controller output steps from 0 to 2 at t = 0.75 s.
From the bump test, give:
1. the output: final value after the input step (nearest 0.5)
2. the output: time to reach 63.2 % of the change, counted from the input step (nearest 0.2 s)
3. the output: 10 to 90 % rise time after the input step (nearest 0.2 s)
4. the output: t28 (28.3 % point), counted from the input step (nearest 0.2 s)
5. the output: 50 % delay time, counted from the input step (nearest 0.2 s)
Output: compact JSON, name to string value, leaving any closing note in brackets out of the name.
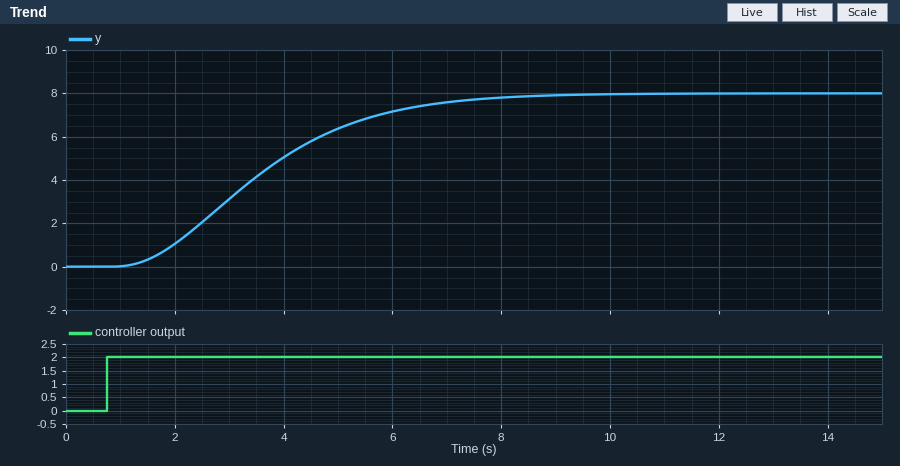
{"the output: final value after the input step": "8.0", "the output: time to reach 63.2 % of the change, counted from the input step": "3.2 s", "the output: 10 to 90 % rise time after the input step": "4.2 s", "the output: t28 (28.3 % point), counted from the input step": "1.8 s", "the output: 50 % delay time, counted from the input step": "2.6 s"}
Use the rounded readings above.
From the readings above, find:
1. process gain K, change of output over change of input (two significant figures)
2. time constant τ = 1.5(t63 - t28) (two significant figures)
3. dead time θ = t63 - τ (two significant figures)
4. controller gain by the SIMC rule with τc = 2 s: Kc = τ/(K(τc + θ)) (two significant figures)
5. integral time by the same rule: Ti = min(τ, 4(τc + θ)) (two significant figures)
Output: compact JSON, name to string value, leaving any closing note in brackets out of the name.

{"process gain K, change of output over change of input": "4.0", "time constant τ = 1.5(t63 - t28)": "2.1 s", "dead time θ = t63 - τ": "1.1 s", "controller gain by the SIMC rule with τc = 2 s: Kc = τ/(K(τc + θ))": "0.17", "integral time by the same rule: Ti = min(τ, 4(τc + θ))": "2.1 s"}
